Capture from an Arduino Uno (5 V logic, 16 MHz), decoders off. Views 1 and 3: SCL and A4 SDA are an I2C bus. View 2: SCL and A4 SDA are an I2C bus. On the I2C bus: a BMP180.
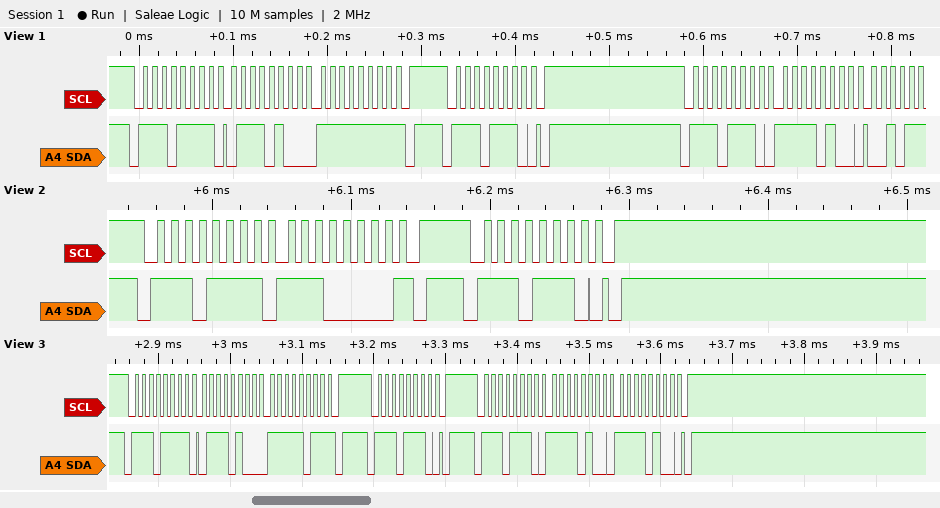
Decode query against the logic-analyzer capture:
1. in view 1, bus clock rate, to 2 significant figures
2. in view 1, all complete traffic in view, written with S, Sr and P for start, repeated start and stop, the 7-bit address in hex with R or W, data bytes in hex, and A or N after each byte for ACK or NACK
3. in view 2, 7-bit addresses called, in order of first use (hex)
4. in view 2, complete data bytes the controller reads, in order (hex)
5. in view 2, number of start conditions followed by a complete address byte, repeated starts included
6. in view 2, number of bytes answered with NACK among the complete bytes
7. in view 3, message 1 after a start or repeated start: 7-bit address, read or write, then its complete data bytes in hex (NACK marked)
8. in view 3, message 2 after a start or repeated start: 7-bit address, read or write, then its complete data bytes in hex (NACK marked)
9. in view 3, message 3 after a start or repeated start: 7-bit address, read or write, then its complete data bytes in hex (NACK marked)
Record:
100 kHz
S 77R A 74 A FF N P S 77W A P S 77W A F4 A
0x77
E0
2
1
0x77 read: 74 FB NACK
0x77 write
0x77 write: F4 F4
